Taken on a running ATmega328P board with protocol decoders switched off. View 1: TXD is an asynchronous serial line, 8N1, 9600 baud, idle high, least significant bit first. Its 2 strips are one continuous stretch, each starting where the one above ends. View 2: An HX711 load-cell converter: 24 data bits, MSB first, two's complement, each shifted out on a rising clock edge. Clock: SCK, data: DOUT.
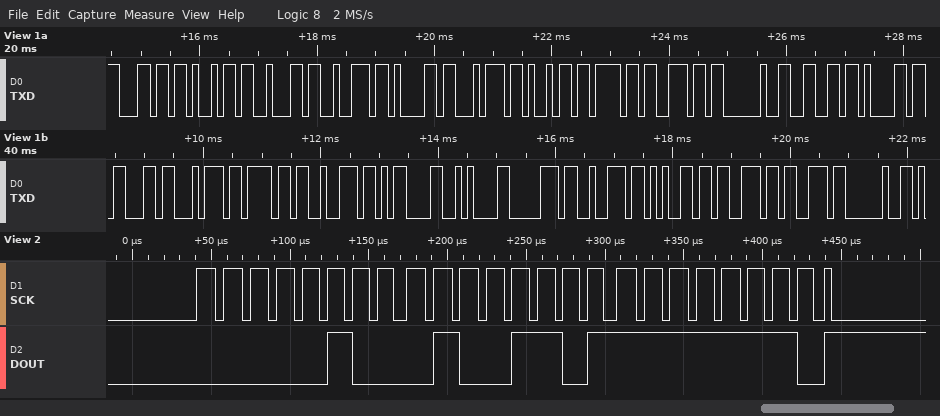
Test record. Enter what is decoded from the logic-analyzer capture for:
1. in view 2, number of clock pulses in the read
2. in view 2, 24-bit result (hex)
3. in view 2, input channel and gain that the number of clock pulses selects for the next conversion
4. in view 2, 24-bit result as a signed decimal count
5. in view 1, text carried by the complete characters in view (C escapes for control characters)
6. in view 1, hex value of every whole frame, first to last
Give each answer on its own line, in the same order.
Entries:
25
0x044DFE
channel A, gain 128
282110
"libration factor\r\npress "
6C 69 62 72 61 74 69 6F 6E 20 66 61 63 74 6F 72 0D 0A 70 72 65 73 73 20
